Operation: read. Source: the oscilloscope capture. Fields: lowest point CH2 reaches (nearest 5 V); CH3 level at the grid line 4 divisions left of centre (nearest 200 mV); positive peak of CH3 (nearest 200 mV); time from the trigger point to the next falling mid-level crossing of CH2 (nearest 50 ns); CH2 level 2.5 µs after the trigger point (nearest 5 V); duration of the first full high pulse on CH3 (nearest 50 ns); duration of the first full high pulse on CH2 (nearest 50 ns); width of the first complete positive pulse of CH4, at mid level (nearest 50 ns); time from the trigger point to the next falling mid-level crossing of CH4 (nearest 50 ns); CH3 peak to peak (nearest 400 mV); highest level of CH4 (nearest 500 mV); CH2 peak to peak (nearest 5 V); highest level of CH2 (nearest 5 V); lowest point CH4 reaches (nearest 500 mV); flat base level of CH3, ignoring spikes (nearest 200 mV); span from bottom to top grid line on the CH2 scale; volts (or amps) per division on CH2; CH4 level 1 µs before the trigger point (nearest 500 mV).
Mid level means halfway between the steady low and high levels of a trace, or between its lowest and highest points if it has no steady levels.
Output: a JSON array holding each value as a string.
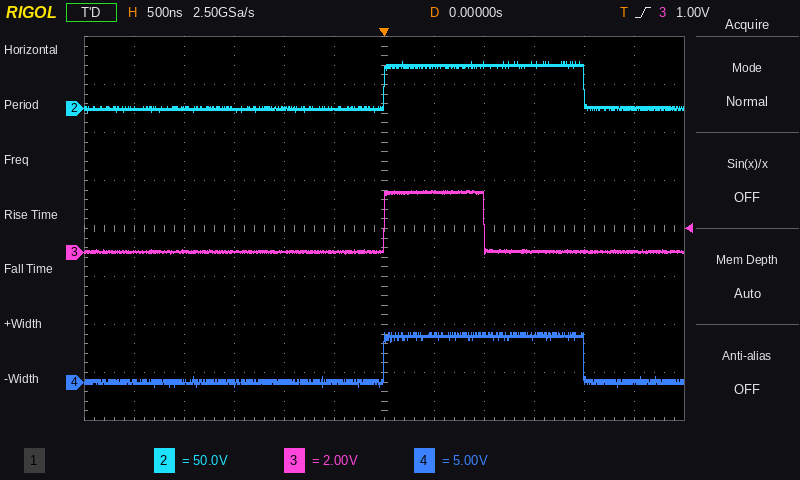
["-5 V", "0.0 V", "2.6 V", "2.00 µs", "0 V", "1.00 µs", "2.00 µs", "2.00 µs", "2.00 µs", "2.8 V", "5.0 V", "55 V", "50 V", "-500 mV", "0.0 V", "400 V", "50 V", "0.0 V"]
